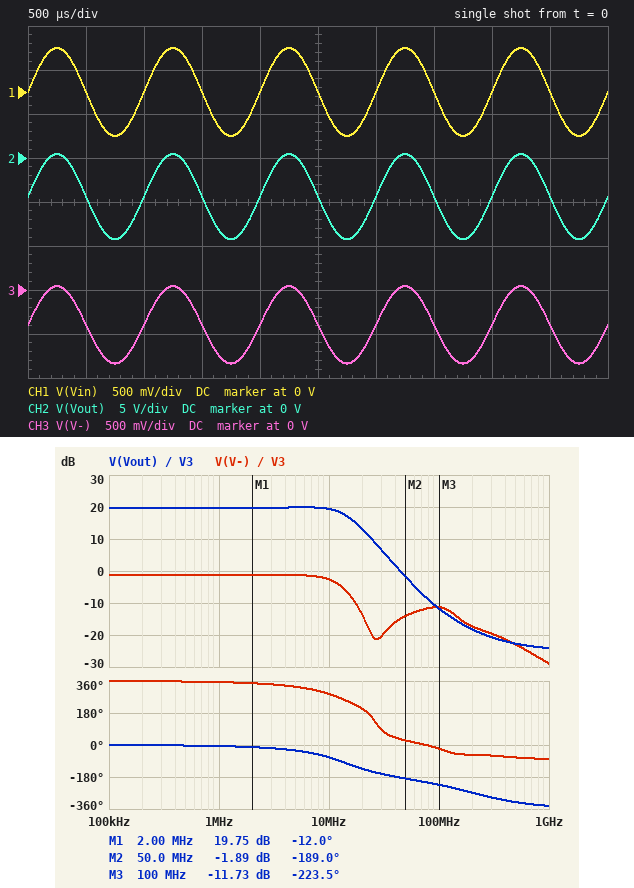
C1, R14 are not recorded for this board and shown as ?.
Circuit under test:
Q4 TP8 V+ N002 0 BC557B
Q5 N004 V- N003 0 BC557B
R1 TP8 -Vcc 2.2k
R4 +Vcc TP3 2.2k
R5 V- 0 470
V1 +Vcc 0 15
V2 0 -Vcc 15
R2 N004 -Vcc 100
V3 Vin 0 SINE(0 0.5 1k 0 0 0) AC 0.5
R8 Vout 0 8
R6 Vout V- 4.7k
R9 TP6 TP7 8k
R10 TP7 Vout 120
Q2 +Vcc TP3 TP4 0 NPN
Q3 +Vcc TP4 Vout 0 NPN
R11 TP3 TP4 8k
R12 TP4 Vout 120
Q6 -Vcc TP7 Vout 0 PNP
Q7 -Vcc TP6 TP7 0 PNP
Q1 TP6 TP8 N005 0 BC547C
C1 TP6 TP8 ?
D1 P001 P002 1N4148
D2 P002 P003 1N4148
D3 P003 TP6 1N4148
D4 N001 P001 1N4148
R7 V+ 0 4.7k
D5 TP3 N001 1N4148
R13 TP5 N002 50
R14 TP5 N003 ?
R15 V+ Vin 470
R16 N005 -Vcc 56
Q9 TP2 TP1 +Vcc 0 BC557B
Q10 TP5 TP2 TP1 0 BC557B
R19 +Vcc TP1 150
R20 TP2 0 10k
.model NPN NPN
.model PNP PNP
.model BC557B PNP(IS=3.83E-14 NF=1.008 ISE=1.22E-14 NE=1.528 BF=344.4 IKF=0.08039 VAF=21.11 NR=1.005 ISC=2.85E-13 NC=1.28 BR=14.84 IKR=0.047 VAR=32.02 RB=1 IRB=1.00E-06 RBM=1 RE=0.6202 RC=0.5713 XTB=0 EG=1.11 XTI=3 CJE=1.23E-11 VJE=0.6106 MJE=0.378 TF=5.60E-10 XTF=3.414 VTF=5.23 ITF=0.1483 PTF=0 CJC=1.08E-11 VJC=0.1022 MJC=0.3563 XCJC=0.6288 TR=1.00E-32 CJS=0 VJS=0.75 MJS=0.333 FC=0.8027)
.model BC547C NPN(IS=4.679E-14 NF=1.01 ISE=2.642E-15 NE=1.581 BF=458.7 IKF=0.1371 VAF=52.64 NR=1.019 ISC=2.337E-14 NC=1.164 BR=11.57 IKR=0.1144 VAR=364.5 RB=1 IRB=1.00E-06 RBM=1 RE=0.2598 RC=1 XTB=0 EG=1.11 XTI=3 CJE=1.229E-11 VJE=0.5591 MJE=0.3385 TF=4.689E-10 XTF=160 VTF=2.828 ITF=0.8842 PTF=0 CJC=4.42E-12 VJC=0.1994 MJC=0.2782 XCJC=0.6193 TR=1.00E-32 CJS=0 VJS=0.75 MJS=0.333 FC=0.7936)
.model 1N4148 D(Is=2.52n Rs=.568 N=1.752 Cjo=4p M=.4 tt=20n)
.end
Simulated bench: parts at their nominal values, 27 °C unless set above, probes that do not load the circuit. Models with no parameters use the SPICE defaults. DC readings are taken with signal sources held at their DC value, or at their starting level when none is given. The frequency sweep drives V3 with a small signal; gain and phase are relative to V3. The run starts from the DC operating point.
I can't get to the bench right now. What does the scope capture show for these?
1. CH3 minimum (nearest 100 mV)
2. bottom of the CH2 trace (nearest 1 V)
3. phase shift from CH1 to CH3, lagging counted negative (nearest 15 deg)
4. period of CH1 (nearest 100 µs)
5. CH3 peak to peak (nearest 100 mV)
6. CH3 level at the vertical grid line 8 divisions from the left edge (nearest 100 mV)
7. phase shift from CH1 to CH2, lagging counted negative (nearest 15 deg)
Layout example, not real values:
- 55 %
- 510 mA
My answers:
- -800 mV
- -9 V
- 0 deg
- 1.0 ms
- 900 mV
- -400 mV
- 0 deg
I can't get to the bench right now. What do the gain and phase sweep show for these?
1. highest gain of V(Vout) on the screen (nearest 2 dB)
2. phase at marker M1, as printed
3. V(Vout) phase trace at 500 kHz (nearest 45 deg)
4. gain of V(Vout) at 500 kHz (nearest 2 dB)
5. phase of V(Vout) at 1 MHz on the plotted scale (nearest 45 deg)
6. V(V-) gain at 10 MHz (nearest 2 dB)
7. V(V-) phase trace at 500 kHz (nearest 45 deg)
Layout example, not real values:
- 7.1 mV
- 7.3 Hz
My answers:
- 20 dB
- -12.0 deg
- 0 deg
- 20 dB
- 0 deg
- -2 dB
- 360 deg
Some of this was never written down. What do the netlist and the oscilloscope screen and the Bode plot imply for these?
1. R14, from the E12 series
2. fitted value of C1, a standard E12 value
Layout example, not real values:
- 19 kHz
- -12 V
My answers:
- 100 Ω
- 4.7 pF
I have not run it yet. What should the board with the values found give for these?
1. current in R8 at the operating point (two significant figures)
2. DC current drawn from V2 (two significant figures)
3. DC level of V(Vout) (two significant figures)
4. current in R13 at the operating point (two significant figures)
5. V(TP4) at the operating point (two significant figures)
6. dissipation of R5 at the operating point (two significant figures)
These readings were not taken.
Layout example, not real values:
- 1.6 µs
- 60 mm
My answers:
- 550 mA
- 570 mA
- -4.4 V
- 530 µA
- -3.6 V
- 330 µW
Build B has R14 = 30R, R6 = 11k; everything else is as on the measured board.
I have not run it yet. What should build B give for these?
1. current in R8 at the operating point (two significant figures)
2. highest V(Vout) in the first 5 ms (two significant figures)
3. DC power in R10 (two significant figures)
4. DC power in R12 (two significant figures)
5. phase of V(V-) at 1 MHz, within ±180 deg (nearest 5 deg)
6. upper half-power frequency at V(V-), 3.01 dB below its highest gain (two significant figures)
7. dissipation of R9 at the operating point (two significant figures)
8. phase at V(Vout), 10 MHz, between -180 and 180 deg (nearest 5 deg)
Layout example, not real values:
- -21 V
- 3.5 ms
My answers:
- 430 mA
- 7.1 V
- 7.2 mW
- 5.4 mW
- -10 deg
- 7.7 MHz
- 88 µW
- -100 deg
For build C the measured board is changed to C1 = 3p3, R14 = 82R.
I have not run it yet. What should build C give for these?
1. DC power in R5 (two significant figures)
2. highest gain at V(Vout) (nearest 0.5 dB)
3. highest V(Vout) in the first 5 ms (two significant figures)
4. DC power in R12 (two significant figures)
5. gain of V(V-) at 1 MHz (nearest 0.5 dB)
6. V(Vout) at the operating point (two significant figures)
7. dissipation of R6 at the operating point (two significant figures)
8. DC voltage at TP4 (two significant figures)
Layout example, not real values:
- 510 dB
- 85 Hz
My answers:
- 230 µW
- 21.0 dB
- 1.2 V
- 5.4 mW
- -1.0 dB
- -3.7 V
- 2.4 mW
- -2.9 V
